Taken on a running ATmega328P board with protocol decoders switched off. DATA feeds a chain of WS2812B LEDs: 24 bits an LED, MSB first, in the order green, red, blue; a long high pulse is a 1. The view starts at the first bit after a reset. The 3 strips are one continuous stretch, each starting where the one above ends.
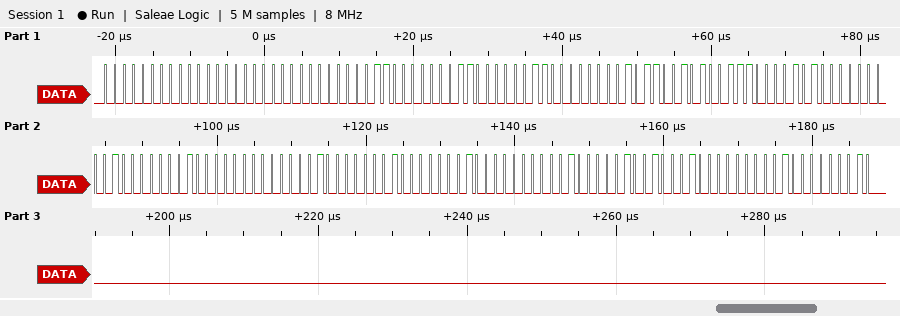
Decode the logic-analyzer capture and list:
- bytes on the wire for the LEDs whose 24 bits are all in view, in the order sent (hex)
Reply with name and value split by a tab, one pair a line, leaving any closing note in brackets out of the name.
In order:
bytes on the wire for the LEDs whose 24 bits are all in view, in the order sent	00 00 00 06 03 03 00 B2 9C 28 02 02 00 08 08 08 01 04 88 02 02
